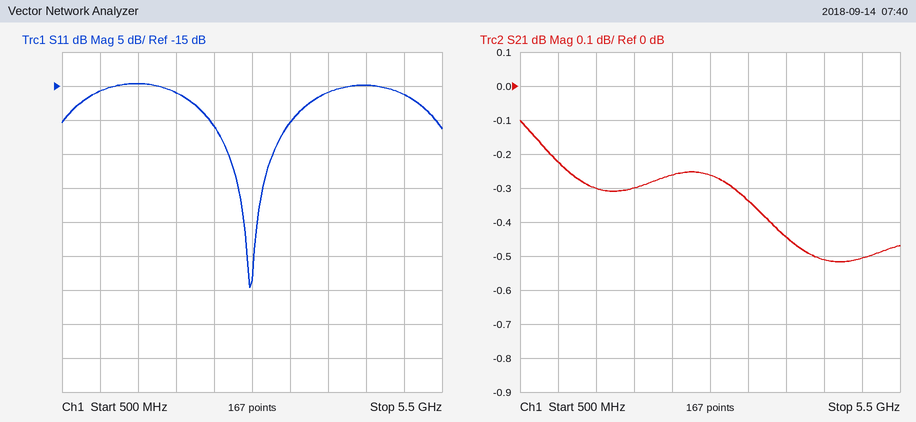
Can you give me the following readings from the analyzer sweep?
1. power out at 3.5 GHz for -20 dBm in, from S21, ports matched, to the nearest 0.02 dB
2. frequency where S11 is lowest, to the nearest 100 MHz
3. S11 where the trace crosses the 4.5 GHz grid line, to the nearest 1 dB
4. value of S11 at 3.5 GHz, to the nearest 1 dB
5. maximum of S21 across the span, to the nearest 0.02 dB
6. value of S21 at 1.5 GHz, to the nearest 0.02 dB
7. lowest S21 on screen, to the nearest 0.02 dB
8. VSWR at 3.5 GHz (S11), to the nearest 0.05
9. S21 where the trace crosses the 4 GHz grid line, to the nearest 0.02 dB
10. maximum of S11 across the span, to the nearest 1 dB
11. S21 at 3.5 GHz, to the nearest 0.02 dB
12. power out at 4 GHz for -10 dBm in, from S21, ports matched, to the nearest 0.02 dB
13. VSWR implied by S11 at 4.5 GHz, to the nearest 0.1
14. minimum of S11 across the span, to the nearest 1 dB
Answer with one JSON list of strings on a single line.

["-20.34 dBm", "3.0 GHz", "-15 dB", "-20 dB", "-0.10 dB", "-0.30 dB", "-0.52 dB", "1.20", "-0.44 dB", "-15 dB", "-0.34 dB", "-10.44 dBm", "1.4", "-45 dB"]
